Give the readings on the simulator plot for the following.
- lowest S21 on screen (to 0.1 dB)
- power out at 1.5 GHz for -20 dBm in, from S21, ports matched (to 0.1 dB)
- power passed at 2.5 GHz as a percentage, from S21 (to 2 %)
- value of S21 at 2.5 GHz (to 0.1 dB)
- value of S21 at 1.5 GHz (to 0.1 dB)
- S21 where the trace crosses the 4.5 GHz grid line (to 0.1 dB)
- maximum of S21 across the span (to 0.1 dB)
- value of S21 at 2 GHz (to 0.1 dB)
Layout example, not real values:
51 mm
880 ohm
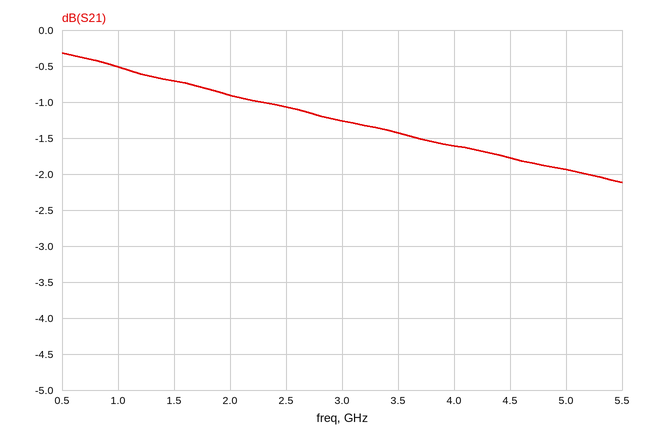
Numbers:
-2.1 dB
-20.7 dBm
78 %
-1.1 dB
-0.7 dB
-1.8 dB
-0.3 dB
-0.9 dB
